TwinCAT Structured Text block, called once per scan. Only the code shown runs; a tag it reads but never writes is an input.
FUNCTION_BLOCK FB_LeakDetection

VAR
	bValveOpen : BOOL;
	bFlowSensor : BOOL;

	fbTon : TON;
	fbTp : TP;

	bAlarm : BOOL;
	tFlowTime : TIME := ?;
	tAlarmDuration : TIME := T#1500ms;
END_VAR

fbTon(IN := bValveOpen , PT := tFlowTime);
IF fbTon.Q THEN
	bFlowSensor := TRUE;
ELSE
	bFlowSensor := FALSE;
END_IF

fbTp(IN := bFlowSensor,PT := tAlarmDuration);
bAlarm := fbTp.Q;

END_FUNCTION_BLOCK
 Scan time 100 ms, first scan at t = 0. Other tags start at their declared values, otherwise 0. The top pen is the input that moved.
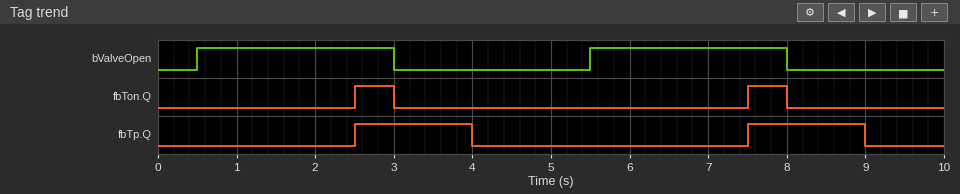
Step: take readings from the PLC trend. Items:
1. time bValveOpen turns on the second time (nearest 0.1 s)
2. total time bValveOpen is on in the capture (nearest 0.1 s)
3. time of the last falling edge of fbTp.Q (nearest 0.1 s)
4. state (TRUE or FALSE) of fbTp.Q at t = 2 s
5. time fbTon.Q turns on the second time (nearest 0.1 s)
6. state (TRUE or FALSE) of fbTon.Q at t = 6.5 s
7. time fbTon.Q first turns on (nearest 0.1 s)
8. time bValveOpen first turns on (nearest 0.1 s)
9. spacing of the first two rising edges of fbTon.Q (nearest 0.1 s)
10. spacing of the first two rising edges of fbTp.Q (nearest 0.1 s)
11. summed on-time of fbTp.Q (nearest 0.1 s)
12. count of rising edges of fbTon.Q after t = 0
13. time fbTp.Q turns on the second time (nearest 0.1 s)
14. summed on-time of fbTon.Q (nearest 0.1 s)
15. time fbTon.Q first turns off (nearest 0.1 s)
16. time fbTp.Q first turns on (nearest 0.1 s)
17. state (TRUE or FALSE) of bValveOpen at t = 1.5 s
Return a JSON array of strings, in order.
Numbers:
["5.5 s", "5.0 s", "9.0 s", "FALSE", "7.5 s", "FALSE", "2.5 s", "0.5 s", "5.0 s", "5.0 s", "3.0 s", "2", "7.5 s", "1.0 s", "3.0 s", "2.5 s", "TRUE"]
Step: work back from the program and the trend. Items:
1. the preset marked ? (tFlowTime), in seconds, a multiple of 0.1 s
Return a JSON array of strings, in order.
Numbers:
["2.0 s"]
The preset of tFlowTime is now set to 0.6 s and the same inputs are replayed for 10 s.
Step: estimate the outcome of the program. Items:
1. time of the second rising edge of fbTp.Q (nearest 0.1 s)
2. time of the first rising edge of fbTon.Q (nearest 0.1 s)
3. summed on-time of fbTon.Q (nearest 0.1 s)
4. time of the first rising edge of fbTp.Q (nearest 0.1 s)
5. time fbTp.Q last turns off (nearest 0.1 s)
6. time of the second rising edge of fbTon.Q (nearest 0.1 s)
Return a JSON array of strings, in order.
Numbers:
["6.1 s", "1.1 s", "3.8 s", "1.1 s", "7.6 s", "6.1 s"]
